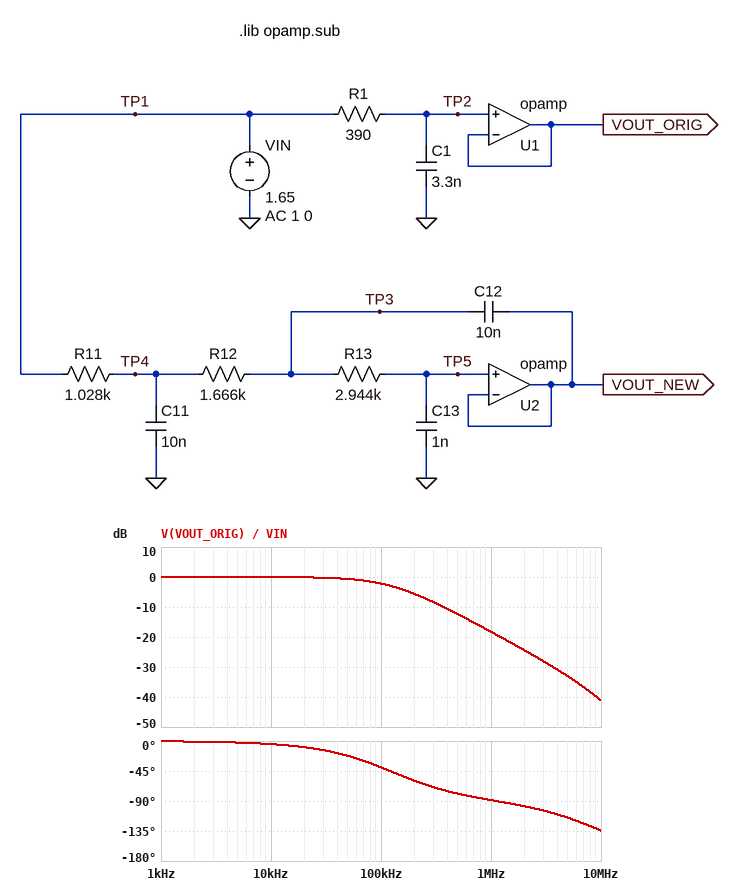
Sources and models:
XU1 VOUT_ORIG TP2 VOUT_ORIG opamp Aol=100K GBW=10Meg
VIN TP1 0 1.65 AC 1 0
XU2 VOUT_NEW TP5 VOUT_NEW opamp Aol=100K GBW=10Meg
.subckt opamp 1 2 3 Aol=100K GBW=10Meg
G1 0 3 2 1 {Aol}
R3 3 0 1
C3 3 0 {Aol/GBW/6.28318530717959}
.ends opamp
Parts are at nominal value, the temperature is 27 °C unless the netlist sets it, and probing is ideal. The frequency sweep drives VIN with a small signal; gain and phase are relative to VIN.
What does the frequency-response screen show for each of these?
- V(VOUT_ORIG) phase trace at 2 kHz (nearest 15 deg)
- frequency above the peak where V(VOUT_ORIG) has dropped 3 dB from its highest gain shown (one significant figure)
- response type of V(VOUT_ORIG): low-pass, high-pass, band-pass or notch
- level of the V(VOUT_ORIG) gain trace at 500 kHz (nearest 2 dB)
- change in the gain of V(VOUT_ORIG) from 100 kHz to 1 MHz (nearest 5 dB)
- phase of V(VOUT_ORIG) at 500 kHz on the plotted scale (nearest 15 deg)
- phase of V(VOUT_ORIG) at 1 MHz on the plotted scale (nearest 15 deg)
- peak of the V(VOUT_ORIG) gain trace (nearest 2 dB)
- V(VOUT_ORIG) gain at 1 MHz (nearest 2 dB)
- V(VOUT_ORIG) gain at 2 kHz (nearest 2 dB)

0 deg
100 kHz
low-pass
-12 dB
-15 dB
-75 deg
-90 deg
0 dB
-18 dB
0 dB
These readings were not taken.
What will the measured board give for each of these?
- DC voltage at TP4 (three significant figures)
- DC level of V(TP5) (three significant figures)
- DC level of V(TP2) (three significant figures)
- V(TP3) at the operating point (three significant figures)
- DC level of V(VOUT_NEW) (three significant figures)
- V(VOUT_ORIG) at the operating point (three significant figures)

1.65 V
1.65 V
1.65 V
1.65 V
1.65 V
1.65 V
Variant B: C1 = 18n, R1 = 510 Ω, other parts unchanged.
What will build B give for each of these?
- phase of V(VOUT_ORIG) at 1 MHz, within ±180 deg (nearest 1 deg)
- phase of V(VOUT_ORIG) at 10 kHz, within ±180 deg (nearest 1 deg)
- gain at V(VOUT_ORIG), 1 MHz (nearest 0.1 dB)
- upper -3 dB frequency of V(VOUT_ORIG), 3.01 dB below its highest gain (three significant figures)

-95 deg
-30 deg
-35.3 dB
17.3 kHz
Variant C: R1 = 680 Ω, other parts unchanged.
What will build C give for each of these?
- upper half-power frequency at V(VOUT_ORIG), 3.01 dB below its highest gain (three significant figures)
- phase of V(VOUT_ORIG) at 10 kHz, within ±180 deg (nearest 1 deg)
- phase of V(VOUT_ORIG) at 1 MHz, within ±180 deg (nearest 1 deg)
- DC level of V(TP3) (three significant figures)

70.9 kHz
-8 deg
-92 deg
1.65 V
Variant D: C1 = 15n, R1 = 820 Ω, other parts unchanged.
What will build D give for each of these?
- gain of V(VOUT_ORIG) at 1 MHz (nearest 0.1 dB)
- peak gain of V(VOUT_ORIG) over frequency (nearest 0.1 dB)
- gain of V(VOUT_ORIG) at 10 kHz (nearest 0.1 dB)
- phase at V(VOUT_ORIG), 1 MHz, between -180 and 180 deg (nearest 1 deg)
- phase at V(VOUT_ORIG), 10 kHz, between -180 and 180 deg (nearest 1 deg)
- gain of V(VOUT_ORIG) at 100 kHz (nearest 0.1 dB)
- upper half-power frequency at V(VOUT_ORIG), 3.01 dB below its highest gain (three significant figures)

-37.8 dB
0 dB
-2.0 dB
-95 deg
-38 deg
-17.8 dB
12.9 kHz
